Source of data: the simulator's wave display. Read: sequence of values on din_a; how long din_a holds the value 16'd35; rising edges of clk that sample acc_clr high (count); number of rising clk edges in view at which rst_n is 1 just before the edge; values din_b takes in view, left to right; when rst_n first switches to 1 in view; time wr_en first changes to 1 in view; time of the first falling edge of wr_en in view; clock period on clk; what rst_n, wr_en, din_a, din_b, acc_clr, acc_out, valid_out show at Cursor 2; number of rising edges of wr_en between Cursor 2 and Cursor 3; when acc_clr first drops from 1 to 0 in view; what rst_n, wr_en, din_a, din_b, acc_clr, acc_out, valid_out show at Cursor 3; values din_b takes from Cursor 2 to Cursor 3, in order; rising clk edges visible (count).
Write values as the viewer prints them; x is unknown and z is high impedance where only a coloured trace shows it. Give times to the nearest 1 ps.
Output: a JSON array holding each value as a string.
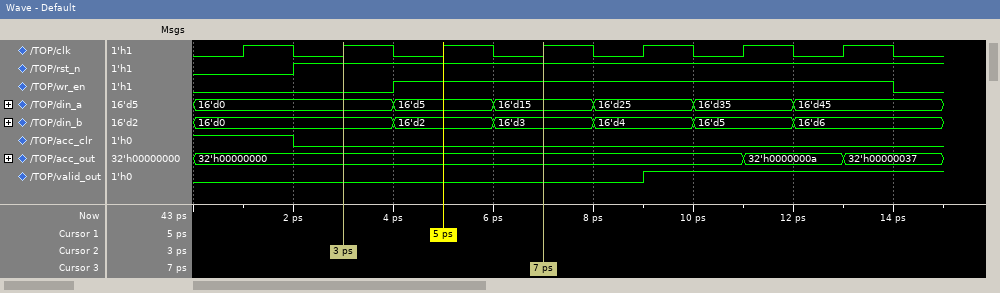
["16'd0, 16'd5, 16'd15, 16'd25, 16'd35, 16'd45", "2 ps", "1", "6", "16'd0, 16'd2, 16'd3, 16'd4, 16'd5, 16'd6", "2 ps", "4 ps", "14 ps", "2 ps", "rst_n=1, wr_en=0, din_a=16'd0, din_b=16'd0, acc_clr=0, acc_out=32'h00000000, valid_out=0", "1", "2 ps", "rst_n=1, wr_en=1, din_a=16'd15, din_b=16'd3, acc_clr=0, acc_out=32'h00000000, valid_out=0", "16'd0, 16'd2, 16'd3", "7"]
